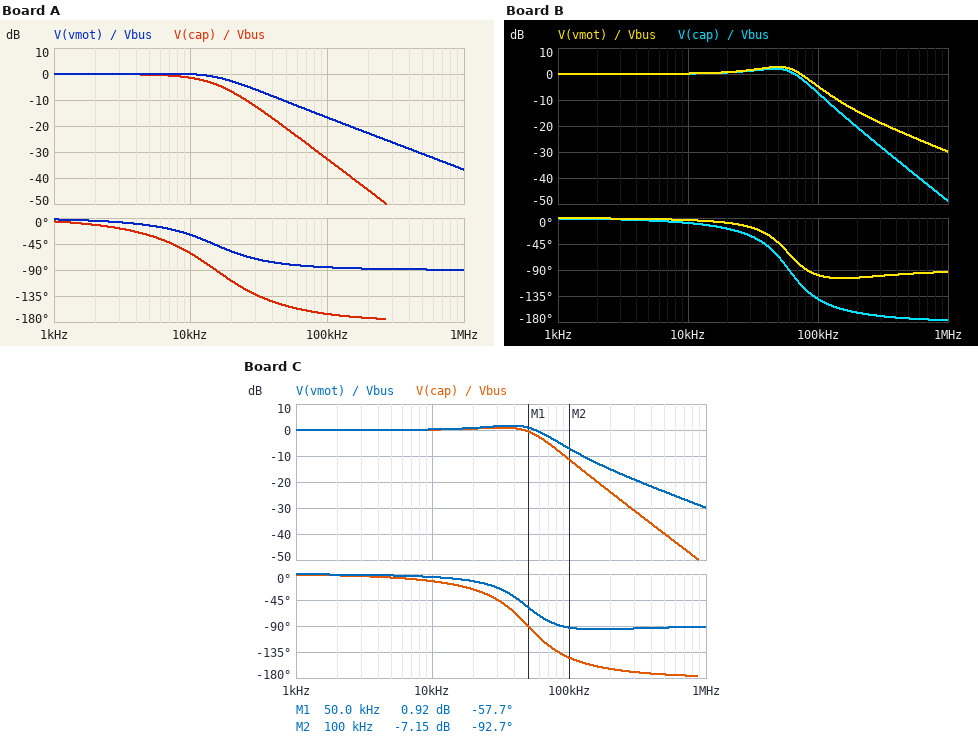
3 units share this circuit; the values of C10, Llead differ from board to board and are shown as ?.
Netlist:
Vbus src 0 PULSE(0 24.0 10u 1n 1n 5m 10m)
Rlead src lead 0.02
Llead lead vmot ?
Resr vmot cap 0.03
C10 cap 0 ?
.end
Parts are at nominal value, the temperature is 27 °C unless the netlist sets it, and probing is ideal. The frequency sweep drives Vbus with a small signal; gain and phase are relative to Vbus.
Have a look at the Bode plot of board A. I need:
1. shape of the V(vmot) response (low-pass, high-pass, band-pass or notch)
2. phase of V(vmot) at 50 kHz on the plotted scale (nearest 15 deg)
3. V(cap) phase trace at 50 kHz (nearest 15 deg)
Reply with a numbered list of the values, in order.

1. low-pass
2. -75 deg
3. -150 deg
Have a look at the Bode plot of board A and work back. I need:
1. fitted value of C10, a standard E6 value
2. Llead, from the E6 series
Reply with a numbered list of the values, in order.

1. 330 µF
2. 330 nH
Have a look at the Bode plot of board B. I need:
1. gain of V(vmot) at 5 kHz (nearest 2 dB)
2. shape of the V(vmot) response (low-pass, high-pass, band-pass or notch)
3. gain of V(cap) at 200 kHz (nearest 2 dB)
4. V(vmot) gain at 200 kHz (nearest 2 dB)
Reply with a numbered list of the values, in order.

1. 0 dB
2. low-pass
3. -20 dB
4. -14 dB
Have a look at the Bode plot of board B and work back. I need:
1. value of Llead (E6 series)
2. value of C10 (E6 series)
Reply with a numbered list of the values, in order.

1. 150 nH
2. 47 µF
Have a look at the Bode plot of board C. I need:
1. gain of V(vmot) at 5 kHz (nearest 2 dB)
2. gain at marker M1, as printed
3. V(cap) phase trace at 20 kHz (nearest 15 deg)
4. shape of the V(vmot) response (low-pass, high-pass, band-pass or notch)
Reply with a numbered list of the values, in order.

1. 0 dB
2. 0.92 dB
3. -30 deg
4. low-pass
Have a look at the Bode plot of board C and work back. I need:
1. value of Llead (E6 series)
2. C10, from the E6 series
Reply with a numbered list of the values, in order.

1. 150 nH
2. 68 µF
